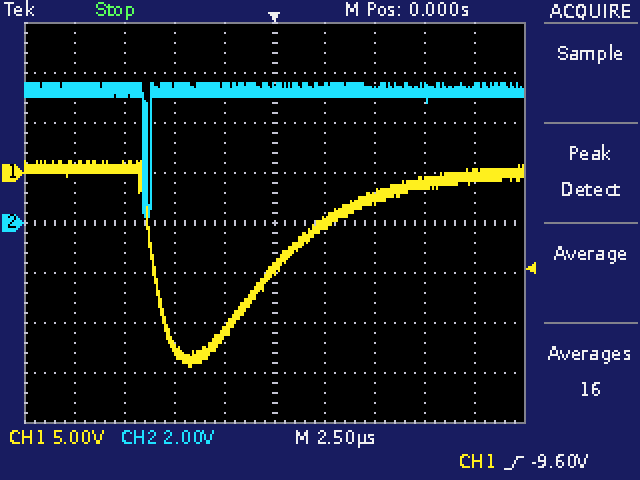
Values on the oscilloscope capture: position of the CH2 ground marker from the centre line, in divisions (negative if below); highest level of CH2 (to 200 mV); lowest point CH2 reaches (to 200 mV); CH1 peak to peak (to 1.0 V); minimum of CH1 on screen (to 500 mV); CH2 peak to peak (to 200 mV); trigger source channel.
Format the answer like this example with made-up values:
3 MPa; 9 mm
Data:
0.0 div; 5.6 V; 200 mV; 21.0 V; -19.5 V; 5.4 V; CH1
